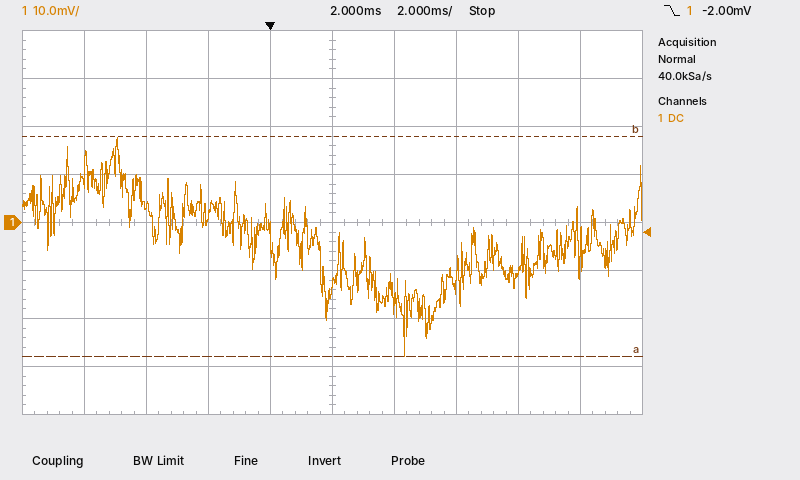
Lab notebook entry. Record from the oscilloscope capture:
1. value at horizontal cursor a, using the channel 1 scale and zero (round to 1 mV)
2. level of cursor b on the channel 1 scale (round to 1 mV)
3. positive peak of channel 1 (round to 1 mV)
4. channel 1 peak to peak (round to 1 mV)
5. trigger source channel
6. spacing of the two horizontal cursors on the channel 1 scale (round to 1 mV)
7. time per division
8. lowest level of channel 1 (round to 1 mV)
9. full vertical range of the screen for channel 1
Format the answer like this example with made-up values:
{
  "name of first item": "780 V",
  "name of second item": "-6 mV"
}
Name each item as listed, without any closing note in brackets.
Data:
{
  "value at horizontal cursor a, using the channel 1 scale and zero": "-28 mV",
  "level of cursor b on the channel 1 scale": "18 mV",
  "positive peak of channel 1": "18 mV",
  "channel 1 peak to peak": "46 mV",
  "trigger source channel": "channel 1",
  "spacing of the two horizontal cursors on the channel 1 scale": "46 mV",
  "time per division": "2 ms",
  "lowest level of channel 1": "-28 mV",
  "full vertical range of the screen for channel 1": "80 mV"
}
